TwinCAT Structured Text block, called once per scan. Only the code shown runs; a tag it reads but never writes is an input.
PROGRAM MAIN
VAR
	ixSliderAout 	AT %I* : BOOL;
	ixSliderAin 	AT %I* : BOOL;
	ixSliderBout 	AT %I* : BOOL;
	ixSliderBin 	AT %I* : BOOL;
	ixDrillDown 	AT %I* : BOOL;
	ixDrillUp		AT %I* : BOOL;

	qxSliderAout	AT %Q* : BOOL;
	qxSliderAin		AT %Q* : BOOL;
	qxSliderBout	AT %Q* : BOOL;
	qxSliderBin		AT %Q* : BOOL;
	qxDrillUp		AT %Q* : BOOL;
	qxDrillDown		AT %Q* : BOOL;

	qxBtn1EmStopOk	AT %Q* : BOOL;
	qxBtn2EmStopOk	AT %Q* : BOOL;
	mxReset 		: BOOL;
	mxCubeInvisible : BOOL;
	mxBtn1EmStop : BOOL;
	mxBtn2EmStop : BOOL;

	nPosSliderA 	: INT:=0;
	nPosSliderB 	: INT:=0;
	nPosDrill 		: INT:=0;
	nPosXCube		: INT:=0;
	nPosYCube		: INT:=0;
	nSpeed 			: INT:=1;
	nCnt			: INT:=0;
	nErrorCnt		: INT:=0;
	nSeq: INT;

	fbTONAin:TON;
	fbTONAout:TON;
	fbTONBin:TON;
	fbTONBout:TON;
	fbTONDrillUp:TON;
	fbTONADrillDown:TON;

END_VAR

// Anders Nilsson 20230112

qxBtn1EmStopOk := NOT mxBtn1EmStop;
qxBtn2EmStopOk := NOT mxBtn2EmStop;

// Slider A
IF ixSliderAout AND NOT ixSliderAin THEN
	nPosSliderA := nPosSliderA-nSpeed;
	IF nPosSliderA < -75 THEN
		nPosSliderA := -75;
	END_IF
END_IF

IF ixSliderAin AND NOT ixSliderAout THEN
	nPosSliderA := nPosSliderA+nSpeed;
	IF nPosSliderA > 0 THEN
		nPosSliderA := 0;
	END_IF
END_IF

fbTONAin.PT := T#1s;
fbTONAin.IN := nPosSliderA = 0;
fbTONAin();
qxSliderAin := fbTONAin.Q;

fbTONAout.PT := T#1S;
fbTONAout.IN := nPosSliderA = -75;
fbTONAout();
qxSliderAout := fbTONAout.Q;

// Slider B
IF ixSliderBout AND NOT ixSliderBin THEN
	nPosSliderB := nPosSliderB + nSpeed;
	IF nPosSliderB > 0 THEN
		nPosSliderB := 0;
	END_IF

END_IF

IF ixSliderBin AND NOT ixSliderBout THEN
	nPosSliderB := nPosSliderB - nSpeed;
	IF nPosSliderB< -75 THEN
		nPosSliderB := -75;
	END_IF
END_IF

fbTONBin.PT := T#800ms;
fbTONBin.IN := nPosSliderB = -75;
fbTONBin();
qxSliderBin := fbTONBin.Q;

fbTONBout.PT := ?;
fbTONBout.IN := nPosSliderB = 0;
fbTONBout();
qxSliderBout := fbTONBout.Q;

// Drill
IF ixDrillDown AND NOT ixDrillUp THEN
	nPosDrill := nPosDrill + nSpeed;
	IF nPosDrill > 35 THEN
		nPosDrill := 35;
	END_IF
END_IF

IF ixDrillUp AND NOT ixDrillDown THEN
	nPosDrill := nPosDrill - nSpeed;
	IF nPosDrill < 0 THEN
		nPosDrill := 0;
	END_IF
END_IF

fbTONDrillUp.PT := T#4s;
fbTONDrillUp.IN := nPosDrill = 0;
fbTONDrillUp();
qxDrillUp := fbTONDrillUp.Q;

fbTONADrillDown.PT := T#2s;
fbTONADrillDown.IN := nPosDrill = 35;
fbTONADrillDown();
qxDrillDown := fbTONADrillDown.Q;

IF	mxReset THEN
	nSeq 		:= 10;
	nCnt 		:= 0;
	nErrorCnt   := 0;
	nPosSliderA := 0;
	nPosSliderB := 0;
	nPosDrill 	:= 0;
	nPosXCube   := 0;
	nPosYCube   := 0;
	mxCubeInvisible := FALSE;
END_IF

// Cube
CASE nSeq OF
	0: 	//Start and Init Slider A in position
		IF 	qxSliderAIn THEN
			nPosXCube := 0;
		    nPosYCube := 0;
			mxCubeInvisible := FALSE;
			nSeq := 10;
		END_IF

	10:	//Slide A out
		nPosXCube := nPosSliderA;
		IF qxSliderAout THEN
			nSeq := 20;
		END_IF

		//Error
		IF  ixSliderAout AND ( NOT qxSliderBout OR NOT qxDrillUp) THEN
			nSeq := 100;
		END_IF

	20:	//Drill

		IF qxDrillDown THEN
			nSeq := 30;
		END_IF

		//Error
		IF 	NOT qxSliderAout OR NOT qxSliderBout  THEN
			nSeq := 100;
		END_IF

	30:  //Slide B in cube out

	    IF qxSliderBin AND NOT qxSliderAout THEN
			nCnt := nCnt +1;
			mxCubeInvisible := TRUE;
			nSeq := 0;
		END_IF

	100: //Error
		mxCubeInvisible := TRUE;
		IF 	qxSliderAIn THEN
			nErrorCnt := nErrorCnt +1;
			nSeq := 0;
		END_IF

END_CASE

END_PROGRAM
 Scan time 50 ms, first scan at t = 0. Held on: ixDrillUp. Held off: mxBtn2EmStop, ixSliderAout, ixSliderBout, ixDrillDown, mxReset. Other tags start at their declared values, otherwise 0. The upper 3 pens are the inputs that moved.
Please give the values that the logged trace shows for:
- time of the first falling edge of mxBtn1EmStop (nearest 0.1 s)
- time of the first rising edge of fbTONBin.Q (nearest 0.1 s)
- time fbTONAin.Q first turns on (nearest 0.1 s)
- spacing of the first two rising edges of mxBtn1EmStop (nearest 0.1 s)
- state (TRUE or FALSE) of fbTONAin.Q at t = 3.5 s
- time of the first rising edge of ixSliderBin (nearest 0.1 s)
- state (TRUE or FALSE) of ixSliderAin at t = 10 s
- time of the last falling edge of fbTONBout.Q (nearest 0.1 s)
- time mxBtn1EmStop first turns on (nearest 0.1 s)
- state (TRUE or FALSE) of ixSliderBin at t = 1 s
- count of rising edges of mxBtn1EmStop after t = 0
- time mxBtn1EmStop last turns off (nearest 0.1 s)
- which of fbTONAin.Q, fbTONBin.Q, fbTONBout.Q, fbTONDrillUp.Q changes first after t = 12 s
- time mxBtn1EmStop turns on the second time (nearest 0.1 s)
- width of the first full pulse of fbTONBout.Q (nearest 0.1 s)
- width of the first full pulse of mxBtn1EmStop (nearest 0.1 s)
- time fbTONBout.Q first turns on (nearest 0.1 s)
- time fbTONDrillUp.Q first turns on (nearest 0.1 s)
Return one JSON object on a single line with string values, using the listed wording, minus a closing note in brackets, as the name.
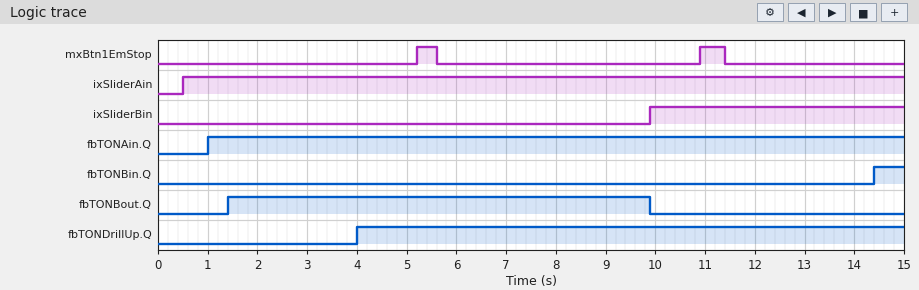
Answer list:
{"time of the first falling edge of mxBtn1EmStop": "5.6 s", "time of the first rising edge of fbTONBin.Q": "14.4 s", "time fbTONAin.Q first turns on": "1.0 s", "spacing of the first two rising edges of mxBtn1EmStop": "5.7 s", "state (TRUE or FALSE) of fbTONAin.Q at t = 3.5 s": "TRUE", "time of the first rising edge of ixSliderBin": "9.9 s", "state (TRUE or FALSE) of ixSliderAin at t = 10 s": "TRUE", "time of the last falling edge of fbTONBout.Q": "9.9 s", "time mxBtn1EmStop first turns on": "5.2 s", "state (TRUE or FALSE) of ixSliderBin at t = 1 s": "FALSE", "count of rising edges of mxBtn1EmStop after t = 0": "2", "time mxBtn1EmStop last turns off": "11.4 s", "which of fbTONAin.Q, fbTONBin.Q, fbTONBout.Q, fbTONDrillUp.Q changes first after t = 12 s": "fbTONBin.Q", "time mxBtn1EmStop turns on the second time": "10.9 s", "width of the first full pulse of fbTONBout.Q": "8.5 s", "width of the first full pulse of mxBtn1EmStop": "0.4 s", "time fbTONBout.Q first turns on": "1.4 s", "time fbTONDrillUp.Q first turns on": "4.0 s"}
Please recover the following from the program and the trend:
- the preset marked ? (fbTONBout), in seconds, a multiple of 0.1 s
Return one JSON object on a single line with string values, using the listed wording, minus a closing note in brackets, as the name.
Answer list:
{"the preset marked ? (fbTONBout), in seconds, a multiple of 0.1 s": "1.4 s"}
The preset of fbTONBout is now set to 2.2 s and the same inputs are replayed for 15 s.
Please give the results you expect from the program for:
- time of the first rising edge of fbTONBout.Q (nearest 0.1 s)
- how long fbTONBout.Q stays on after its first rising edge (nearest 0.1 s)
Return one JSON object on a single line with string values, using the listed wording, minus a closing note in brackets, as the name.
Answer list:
{"time of the first rising edge of fbTONBout.Q": "2.2 s", "how long fbTONBout.Q stays on after its first rising edge": "7.7 s"}
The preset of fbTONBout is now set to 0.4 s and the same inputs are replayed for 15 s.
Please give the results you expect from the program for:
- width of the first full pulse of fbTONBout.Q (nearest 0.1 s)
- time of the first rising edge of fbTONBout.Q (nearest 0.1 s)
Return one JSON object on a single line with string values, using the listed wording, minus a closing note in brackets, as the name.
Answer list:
{"width of the first full pulse of fbTONBout.Q": "9.5 s", "time of the first rising edge of fbTONBout.Q": "0.4 s"}
